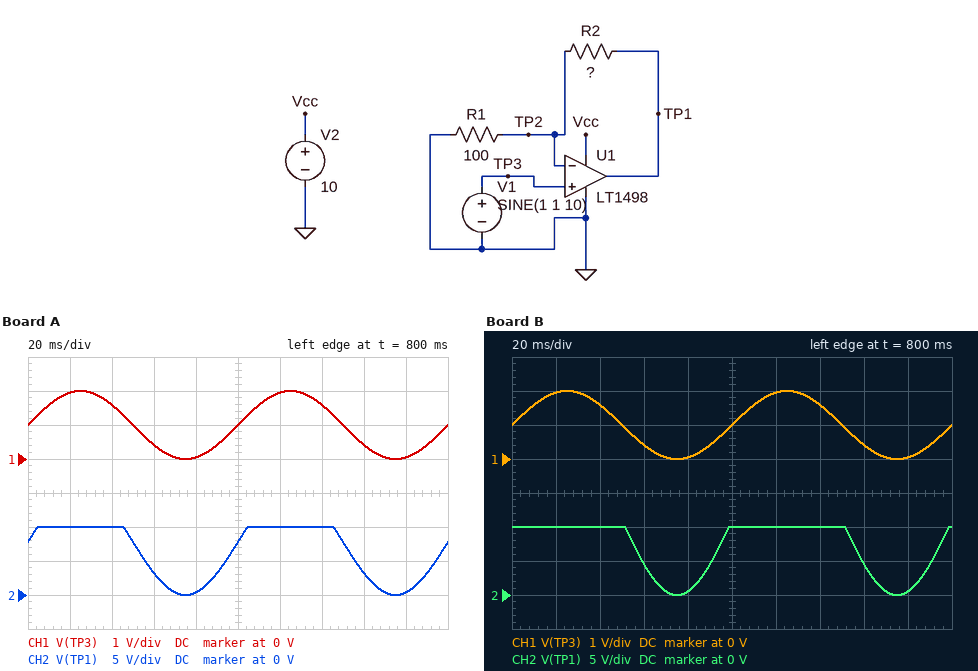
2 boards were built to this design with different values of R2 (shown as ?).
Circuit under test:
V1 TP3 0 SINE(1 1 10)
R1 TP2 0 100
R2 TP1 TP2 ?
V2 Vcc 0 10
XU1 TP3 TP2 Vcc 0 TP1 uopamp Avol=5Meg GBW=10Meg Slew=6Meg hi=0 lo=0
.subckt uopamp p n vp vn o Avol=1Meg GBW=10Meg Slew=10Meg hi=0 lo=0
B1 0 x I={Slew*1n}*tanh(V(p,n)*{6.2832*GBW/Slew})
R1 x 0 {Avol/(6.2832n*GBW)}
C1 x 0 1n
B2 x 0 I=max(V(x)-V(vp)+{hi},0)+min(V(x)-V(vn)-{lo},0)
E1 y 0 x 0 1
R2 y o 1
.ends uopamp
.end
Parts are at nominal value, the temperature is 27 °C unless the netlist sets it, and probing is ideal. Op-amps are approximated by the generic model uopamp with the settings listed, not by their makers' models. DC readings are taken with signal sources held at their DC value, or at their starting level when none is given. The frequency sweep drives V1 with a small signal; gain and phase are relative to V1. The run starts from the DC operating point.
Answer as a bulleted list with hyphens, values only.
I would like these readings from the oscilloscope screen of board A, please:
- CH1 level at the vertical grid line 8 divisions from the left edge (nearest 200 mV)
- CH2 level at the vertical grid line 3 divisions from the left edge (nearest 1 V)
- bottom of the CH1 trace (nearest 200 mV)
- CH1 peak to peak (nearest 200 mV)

- 400 mV
- 3 V
- 0 V
- 2.0 V
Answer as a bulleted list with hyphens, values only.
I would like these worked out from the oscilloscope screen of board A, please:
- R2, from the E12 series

- 680 Ω
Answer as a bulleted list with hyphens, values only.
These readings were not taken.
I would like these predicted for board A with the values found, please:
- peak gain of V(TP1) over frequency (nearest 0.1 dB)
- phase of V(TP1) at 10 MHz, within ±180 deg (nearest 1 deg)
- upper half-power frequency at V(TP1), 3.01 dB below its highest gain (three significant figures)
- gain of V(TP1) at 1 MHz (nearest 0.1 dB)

- 17.8 dB
- -83 deg
- 1.28 MHz
- 15.8 dB
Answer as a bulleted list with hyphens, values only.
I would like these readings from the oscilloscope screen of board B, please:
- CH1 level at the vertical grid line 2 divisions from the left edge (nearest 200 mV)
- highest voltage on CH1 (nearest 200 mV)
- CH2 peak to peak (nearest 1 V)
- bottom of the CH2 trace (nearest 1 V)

- 1.6 V
- 2.0 V
- 10 V
- 0 V
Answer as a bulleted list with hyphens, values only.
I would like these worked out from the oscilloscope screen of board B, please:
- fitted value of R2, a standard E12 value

- 1 kΩ
